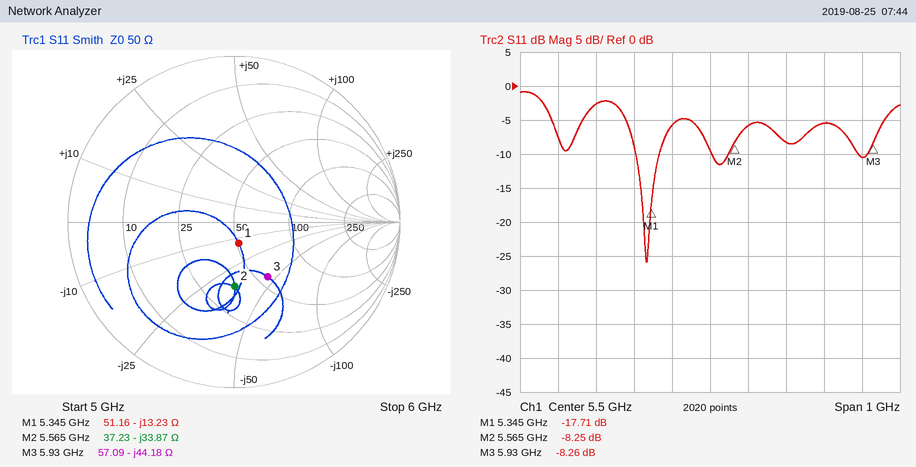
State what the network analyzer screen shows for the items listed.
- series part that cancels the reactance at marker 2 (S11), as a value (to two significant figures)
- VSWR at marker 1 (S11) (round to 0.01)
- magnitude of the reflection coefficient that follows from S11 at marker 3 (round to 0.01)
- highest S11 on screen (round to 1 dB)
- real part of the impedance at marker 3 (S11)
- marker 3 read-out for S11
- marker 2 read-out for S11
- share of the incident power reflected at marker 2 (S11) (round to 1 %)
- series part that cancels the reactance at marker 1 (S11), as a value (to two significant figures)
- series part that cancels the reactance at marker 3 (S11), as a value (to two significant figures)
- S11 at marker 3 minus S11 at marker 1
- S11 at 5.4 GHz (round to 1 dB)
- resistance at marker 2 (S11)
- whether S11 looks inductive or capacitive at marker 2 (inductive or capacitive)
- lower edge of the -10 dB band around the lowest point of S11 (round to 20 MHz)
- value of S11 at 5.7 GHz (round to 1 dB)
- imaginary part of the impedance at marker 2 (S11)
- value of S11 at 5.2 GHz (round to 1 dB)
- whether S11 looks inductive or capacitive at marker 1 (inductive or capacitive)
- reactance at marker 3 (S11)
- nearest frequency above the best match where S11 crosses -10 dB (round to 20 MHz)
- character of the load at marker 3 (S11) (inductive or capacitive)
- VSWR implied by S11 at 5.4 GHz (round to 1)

970 pH
1.30
0.39
-1 dB
57.09 Ω
-8.26 dB
-8.25 dB
15 %
390 pH
1.2 nH
9.45 dB
-6 dB
37.23 Ω
capacitive
5.30 GHz
-8 dB
-33.87 Ω
-3 dB
capacitive
-44.18 Ω
5.36 GHz
capacitive
3
